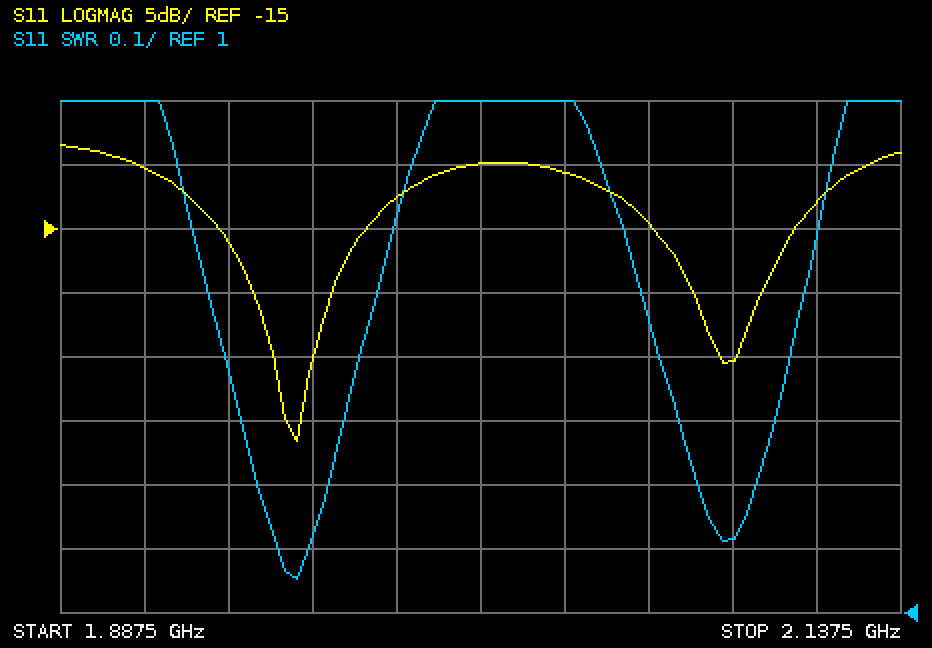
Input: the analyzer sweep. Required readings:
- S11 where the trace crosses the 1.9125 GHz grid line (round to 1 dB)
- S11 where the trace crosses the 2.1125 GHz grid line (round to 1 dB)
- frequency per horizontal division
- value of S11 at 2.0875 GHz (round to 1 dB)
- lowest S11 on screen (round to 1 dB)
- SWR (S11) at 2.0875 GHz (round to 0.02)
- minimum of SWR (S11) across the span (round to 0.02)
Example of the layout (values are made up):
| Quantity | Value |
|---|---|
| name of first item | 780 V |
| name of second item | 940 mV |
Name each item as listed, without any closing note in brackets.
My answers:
| Quantity | Value |
|---|---|
| S11 where the trace crosses the 1.9125 GHz grid line | -10 dB |
| S11 where the trace crosses the 2.1125 GHz grid line | -13 dB |
| frequency per horizontal division | 25 MHz |
| value of S11 at 2.0875 GHz | -25 dB |
| lowest S11 on screen | -32 dB |
| SWR (S11) at 2.0875 GHz | 1.12 |
| minimum of SWR (S11) across the span | 1.06 |
